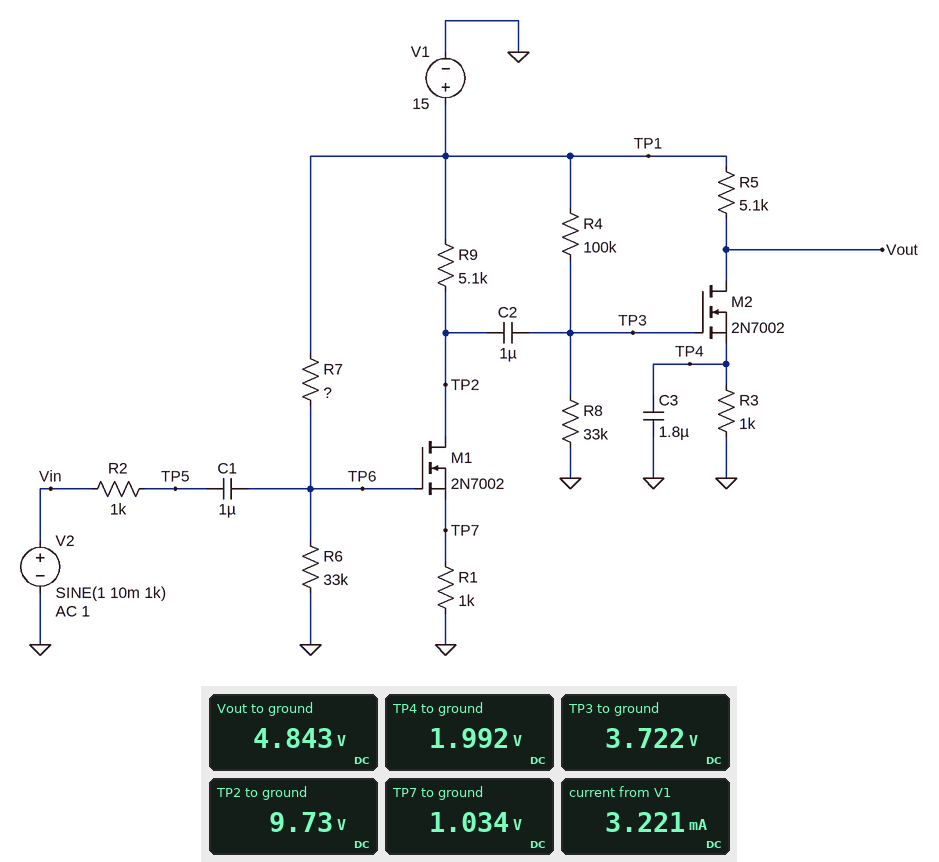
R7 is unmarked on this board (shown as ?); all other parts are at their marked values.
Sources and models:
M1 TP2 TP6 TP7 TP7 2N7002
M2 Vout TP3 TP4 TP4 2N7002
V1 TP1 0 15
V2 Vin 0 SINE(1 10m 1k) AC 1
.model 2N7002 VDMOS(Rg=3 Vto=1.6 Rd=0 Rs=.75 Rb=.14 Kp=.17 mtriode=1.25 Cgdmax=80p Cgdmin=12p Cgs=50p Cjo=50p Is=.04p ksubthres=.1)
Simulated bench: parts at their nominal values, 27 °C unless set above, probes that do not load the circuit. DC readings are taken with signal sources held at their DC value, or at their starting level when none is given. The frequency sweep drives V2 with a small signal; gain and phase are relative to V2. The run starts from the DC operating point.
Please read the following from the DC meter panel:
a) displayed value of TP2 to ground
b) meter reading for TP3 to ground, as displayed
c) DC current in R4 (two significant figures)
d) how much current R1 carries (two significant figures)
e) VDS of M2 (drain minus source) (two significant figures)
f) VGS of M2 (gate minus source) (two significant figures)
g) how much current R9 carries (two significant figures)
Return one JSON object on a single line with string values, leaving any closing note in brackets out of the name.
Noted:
{"displayed value of TP2 to ground": "9.73 V", "meter reading for TP3 to ground, as displayed": "3.722 V", "DC current in R4": "110 µA", "how much current R1 carries": "1.0 mA", "VDS of M2 (drain minus source)": "2.9 V", "VGS of M2 (gate minus source)": "1.7 V", "how much current R9 carries": "1.0 mA"}
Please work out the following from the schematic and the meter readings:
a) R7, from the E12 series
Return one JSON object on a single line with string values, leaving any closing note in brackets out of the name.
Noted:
{"R7, from the E12 series": "150 kΩ"}
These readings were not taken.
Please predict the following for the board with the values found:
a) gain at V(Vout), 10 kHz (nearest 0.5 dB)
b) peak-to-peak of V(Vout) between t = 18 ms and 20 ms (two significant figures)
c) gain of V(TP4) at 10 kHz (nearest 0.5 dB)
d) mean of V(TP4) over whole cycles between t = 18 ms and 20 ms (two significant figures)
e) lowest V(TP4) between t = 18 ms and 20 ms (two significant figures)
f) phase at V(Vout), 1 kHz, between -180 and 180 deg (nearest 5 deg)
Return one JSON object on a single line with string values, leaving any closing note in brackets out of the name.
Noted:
{"gain at V(Vout), 10 kHz": "50.0 dB", "peak-to-peak of V(Vout) between t = 18 ms and 20 ms": "3.8 V", "gain of V(TP4) at 10 kHz": "-5.5 dB", "mean of V(TP4) over whole cycles between t = 18 ms and 20 ms": "2.0 V", "lowest V(TP4) between t = 18 ms and 20 ms": "2.0 V", "phase at V(Vout), 1 kHz, between -180 and 180 deg": "55 deg"}
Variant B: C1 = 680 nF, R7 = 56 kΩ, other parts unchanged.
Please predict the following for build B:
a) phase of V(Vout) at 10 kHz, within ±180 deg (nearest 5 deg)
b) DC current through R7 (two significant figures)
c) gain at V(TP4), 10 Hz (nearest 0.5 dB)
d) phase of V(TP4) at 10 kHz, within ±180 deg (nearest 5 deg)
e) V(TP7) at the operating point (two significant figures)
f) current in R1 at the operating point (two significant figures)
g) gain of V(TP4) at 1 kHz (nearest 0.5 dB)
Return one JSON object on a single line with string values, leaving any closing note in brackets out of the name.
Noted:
{"phase of V(Vout) at 10 kHz, within ±180 deg": "-60 deg", "DC current through R7": "170 µA", "gain at V(TP4), 10 Hz": "-53.0 dB", "phase of V(TP4) at 10 kHz, within ±180 deg": "30 deg", "V(TP7) at the operating point": "2.5 V", "current in R1 at the operating point": "2.5 mA", "gain of V(TP4) at 1 kHz": "-49.5 dB"}
